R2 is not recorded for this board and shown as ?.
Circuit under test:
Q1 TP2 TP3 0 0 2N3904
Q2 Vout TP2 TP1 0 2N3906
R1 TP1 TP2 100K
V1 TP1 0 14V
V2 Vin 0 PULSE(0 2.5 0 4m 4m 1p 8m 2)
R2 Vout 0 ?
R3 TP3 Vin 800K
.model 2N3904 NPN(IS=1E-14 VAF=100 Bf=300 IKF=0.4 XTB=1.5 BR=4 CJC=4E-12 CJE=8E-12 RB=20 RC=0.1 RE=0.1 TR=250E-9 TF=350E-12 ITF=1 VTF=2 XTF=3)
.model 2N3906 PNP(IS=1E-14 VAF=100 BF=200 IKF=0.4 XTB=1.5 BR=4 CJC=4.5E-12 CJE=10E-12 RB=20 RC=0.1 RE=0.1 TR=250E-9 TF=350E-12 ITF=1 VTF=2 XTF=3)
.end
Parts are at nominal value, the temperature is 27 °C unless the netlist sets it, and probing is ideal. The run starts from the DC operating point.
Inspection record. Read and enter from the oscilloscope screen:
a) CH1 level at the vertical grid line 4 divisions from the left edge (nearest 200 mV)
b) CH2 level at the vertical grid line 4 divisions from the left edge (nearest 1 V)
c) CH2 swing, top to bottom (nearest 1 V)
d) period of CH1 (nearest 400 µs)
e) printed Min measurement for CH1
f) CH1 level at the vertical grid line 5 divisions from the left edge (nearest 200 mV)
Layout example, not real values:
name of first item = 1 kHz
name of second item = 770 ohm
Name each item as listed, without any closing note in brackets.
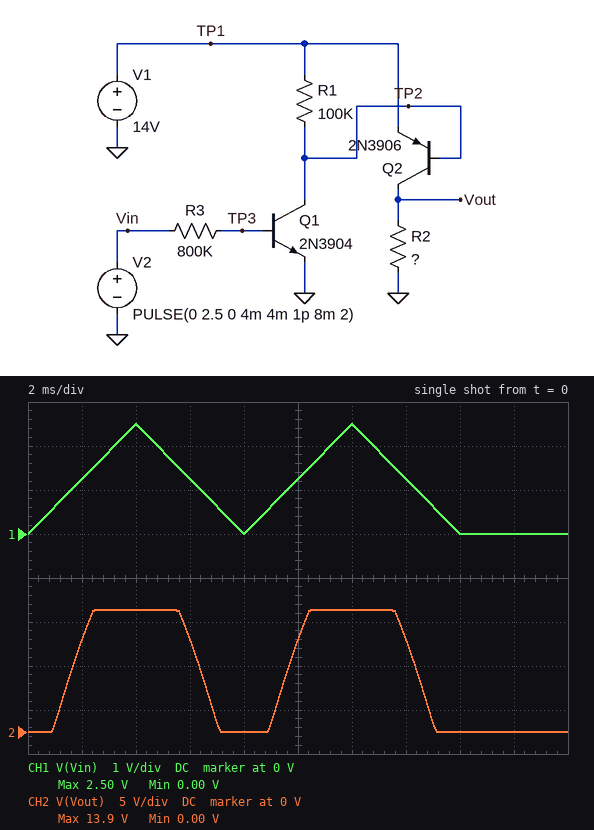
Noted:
CH1 level at the vertical grid line 4 divisions from the left edge = 0 V
CH2 level at the vertical grid line 4 divisions from the left edge = 0 V
CH2 swing, top to bottom = 14 V
period of CH1 = 8.0 ms
printed Min measurement for CH1 = 0.00 V
CH1 level at the vertical grid line 5 divisions from the left edge = 1.2 V
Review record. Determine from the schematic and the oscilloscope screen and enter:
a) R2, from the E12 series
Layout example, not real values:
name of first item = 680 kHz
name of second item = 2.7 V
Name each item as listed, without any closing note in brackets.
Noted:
R2, from the E12 series = 220 Ω
